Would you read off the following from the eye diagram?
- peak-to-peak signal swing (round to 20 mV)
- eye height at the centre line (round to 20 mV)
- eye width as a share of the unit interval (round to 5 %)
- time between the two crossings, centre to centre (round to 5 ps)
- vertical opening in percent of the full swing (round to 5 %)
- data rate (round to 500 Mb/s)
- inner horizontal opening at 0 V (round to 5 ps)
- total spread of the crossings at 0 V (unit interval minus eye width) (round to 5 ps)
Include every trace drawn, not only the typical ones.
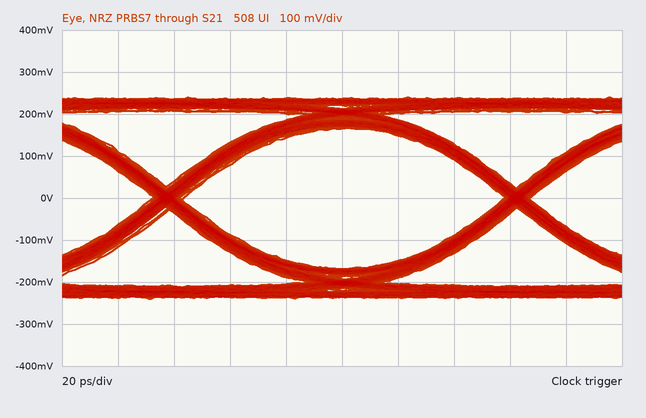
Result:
480 mV
340 mV
90 %
125 ps
70 %
8.0 Gb/s
115 ps
10 ps
